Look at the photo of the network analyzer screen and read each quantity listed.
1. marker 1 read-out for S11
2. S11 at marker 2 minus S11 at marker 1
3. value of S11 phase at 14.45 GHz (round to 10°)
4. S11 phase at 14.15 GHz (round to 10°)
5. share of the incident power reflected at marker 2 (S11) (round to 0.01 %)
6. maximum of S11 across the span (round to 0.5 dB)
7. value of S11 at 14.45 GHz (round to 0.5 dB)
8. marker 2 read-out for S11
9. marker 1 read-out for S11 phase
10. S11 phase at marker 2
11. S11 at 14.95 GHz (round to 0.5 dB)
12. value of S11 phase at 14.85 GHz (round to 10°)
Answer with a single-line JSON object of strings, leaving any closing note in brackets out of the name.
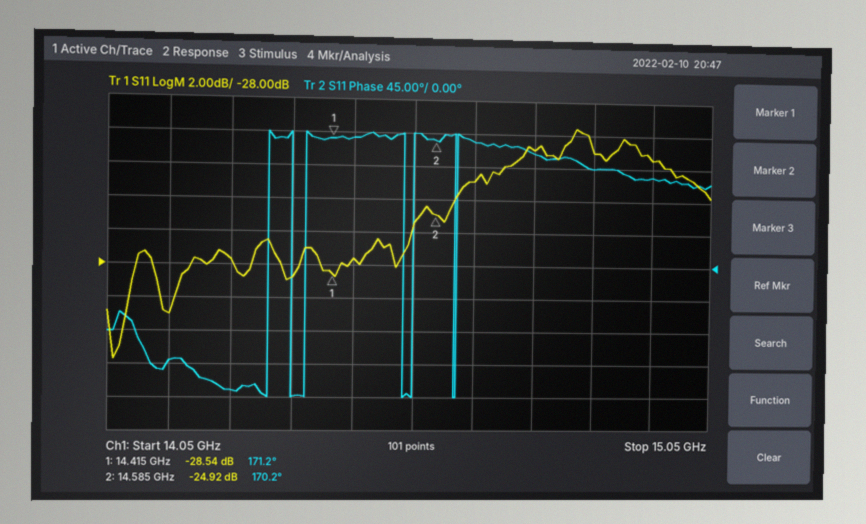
{"marker 1 read-out for S11": "-28.54 dB", "S11 at marker 2 minus S11 at marker 1": "3.62 dB", "value of S11 phase at 14.45 GHz": "170°", "S11 phase at 14.15 GHz": "-130°", "share of the incident power reflected at marker 2 (S11)": "0.32 %", "maximum of S11 across the span": "-19.5 dB", "value of S11 at 14.45 GHz": "-27.5 dB", "marker 2 read-out for S11": "-24.92 dB", "marker 1 read-out for S11 phase": "171.2°", "S11 phase at marker 2": "170.2°", "S11 at 14.95 GHz": "-21.5 dB", "value of S11 phase at 14.85 GHz": "130°"}
